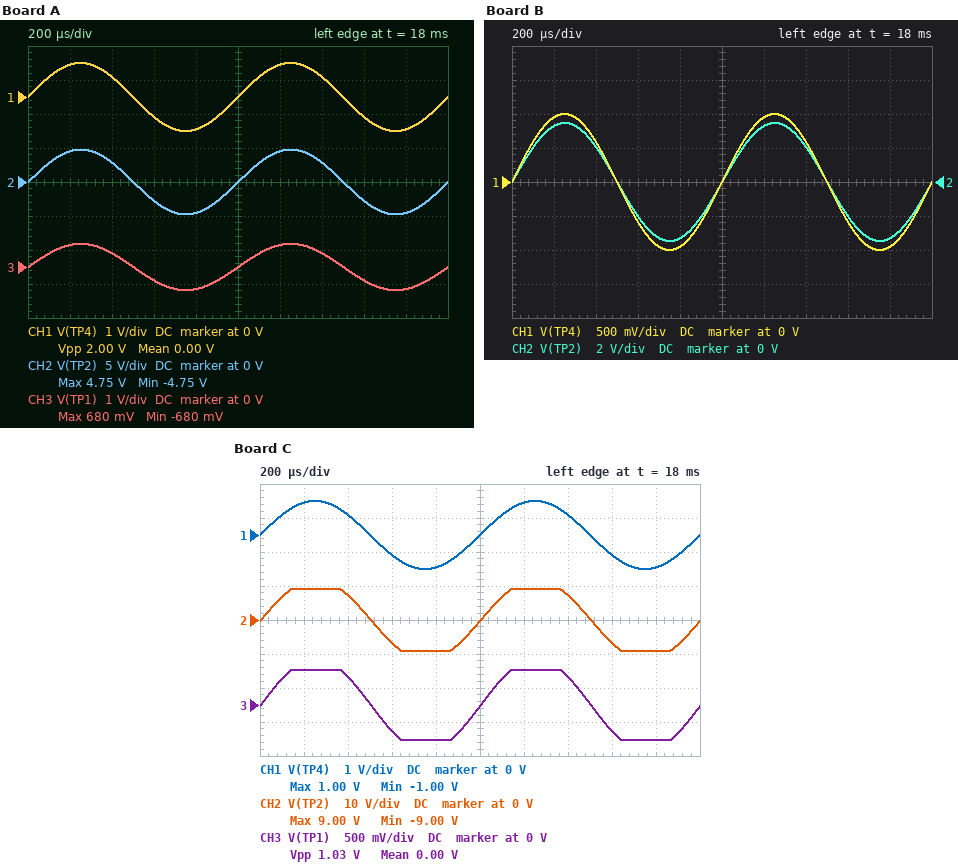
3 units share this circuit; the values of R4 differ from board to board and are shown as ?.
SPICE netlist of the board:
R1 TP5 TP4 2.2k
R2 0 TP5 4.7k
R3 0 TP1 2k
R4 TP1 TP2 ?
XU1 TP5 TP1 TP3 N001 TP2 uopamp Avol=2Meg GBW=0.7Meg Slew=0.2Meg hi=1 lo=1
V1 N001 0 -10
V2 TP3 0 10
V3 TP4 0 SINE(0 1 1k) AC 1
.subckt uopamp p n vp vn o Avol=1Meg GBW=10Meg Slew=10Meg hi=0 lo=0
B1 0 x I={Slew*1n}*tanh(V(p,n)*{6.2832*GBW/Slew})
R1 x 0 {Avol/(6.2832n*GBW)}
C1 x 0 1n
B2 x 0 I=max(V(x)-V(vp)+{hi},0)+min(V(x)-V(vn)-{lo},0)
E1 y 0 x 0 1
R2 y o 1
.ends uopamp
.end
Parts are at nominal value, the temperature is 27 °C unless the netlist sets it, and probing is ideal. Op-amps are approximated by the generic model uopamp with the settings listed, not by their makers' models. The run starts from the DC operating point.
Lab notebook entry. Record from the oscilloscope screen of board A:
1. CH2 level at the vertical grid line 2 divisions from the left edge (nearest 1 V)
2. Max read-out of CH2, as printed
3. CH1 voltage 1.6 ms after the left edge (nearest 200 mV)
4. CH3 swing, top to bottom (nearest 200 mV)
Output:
3 V
4.75 V
-600 mV
1.4 V
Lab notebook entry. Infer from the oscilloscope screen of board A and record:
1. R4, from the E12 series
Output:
12 kΩ
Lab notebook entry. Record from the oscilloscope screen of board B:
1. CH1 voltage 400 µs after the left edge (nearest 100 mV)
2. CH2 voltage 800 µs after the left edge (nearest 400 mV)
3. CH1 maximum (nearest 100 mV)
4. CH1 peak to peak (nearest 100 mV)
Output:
600 mV
-3.2 V
1.0 V
2.0 V
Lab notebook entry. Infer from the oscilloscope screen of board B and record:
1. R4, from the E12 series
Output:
8.2 kΩ
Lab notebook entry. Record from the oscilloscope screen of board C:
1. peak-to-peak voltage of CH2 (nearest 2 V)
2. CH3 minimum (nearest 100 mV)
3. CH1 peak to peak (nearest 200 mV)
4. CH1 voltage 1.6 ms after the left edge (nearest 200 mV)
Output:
18 V
-500 mV
2.0 V
-600 mV
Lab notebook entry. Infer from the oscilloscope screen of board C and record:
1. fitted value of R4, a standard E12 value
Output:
33 kΩ
